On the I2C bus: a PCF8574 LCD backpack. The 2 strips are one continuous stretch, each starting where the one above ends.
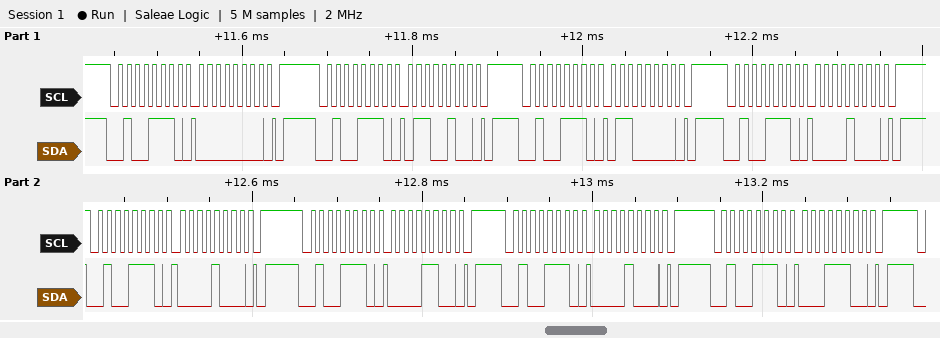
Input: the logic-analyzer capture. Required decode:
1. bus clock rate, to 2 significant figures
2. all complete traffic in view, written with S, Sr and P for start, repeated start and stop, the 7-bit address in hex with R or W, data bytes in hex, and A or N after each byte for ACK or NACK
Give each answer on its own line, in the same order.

100 kHz
S 27W A 00 A P S 27W A 64 A P S 27W A 60 A P S 27W A 08 A P S 27W A 08 A P S 27W A 0C A P S 27W A 08 A P S 27W A 1C A P
